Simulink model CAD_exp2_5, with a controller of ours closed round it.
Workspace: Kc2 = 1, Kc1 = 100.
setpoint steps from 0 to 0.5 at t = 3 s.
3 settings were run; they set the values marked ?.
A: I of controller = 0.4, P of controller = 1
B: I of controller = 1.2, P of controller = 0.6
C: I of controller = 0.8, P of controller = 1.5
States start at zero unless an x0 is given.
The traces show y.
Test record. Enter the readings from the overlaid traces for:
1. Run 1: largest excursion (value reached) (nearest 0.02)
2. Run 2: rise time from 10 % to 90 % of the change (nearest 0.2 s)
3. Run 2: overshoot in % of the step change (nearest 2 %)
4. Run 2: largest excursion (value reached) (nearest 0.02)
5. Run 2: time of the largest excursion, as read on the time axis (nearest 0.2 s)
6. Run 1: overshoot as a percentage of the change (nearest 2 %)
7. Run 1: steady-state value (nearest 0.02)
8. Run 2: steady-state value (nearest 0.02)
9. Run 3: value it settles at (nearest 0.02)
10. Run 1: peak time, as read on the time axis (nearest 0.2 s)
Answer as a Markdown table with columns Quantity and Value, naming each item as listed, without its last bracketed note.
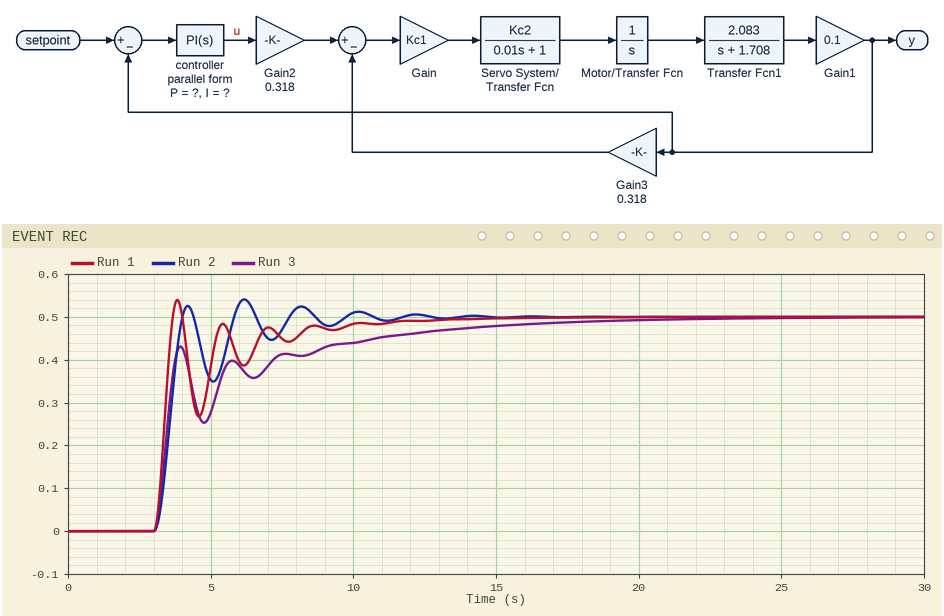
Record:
| Quantity | Value |
|---|---|
| Run 1: largest excursion (value reached) | 0.54 |
| Run 2: rise time from 10 % to 90 % of the change | 0.6 s |
| Run 2: overshoot in % of the step change | 8 % |
| Run 2: largest excursion (value reached) | 0.54 |
| Run 2: time of the largest excursion, as read on the time axis | 6.2 s |
| Run 1: overshoot as a percentage of the change | 8 % |
| Run 1: steady-state value | 0.50 |
| Run 2: steady-state value | 0.50 |
| Run 3: value it settles at | 0.50 |
| Run 1: peak time, as read on the time axis | 3.8 s |
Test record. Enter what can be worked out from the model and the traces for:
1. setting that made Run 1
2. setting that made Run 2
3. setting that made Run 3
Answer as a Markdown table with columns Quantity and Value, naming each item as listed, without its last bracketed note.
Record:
| Quantity | Value |
|---|---|
| setting that made Run 1 | C |
| setting that made Run 2 | B |
| setting that made Run 3 | A |
